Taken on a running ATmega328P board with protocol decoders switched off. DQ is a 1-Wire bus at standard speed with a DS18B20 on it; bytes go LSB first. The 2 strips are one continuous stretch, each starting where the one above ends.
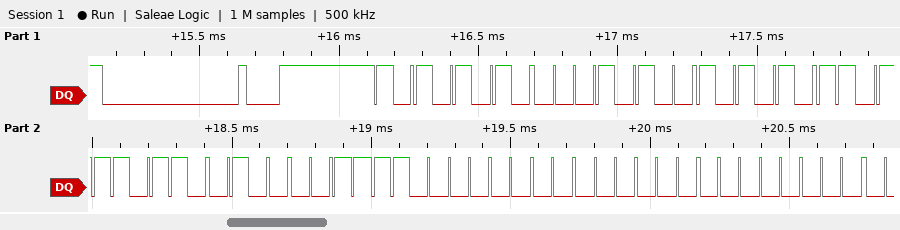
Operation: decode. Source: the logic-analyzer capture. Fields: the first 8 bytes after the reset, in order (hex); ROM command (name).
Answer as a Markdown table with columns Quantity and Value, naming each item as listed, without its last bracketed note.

| Quantity | Value |
|---|---|
| the first 8 bytes after the reset, in order | 55 28 D5 6E C2 03 00 00 |
| ROM command | Match ROM |
